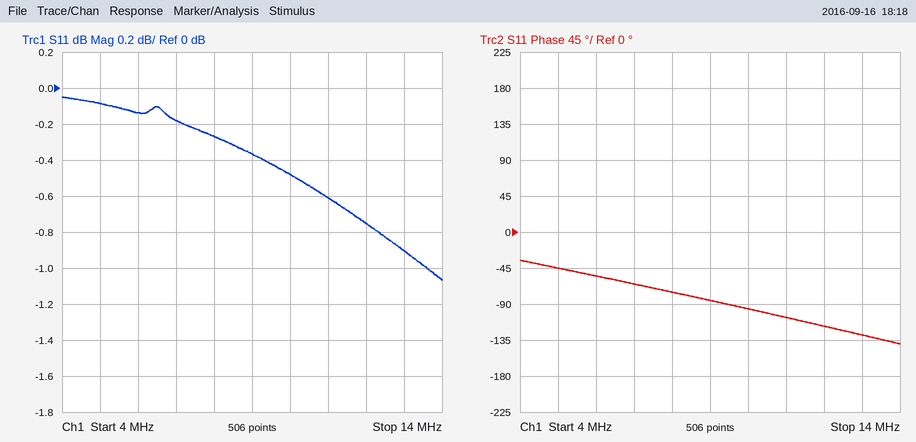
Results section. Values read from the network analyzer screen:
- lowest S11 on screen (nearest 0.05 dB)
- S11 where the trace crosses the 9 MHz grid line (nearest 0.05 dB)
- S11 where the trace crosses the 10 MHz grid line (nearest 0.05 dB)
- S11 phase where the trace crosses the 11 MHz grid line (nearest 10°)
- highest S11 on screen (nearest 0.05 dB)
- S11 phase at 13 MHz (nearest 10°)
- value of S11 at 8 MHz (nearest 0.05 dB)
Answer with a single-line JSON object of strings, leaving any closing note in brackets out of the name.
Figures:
{"lowest S11 on screen": "-1.05 dB", "S11 where the trace crosses the 9 MHz grid line": "-0.35 dB", "S11 where the trace crosses the 10 MHz grid line": "-0.50 dB", "S11 phase where the trace crosses the 11 MHz grid line": "-110°", "highest S11 on screen": "-0.05 dB", "S11 phase at 13 MHz": "-130°", "value of S11 at 8 MHz": "-0.25 dB"}
